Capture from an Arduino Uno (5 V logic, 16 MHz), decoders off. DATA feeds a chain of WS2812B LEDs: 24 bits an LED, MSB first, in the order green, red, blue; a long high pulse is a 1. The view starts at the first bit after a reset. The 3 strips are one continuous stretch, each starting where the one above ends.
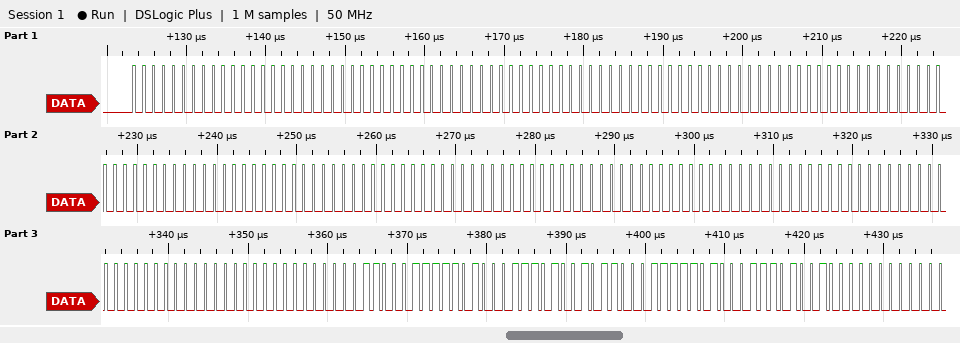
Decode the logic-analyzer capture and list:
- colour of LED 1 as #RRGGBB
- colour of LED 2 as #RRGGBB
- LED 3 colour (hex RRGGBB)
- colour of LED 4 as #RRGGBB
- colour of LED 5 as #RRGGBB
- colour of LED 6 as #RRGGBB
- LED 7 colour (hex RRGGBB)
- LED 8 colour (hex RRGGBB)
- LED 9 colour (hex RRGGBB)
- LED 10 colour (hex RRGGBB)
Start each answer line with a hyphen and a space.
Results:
- #000000
- #000000
- #000000
- #000000
- #000000
- #000000
- #000000
- #000000
- #E863E9
- #E863E9
